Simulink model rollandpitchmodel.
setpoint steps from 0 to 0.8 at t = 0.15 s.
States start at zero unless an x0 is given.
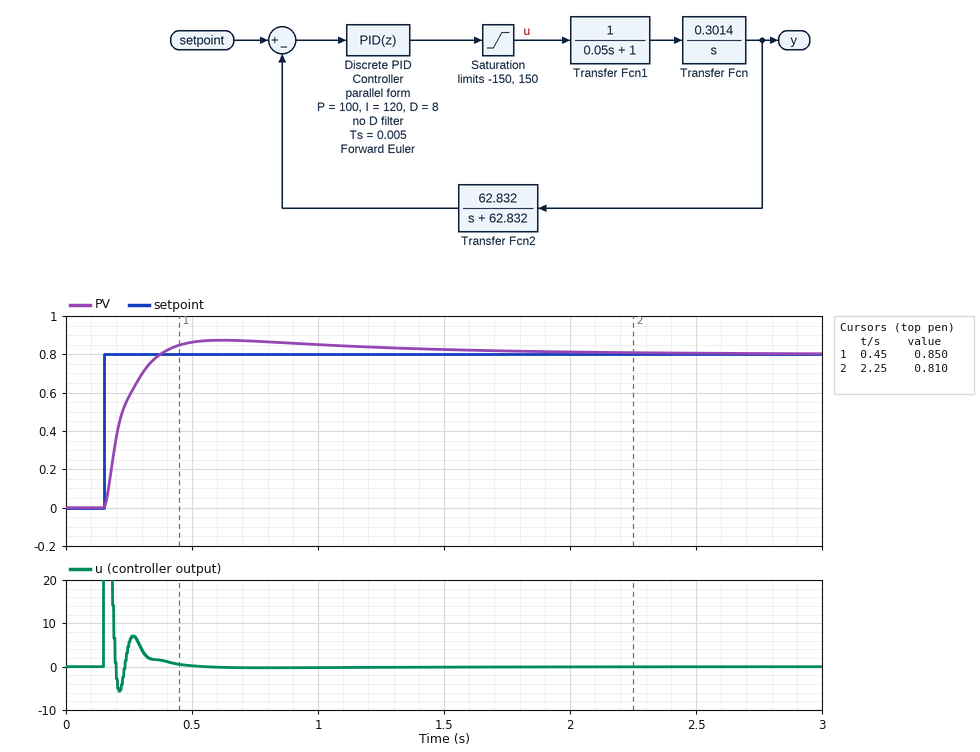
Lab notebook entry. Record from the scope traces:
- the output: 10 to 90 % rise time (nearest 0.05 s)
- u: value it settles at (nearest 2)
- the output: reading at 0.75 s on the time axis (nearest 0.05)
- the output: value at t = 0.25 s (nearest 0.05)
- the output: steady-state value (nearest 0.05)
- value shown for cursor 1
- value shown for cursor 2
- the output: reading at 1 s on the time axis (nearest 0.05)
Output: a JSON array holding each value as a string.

["0.15 s", "0", "0.85", "0.60", "0.80", "0.850", "0.810", "0.85"]
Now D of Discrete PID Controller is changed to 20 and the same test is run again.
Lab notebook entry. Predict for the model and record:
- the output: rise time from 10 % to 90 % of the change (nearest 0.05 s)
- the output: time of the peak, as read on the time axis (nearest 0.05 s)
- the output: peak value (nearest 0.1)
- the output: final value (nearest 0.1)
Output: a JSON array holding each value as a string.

["0.30 s", "1.00 s", "0.9", "0.8"]
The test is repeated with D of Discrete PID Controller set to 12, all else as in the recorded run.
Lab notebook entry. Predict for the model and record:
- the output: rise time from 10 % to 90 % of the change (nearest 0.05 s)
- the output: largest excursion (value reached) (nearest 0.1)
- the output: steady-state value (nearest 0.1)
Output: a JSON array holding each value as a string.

["0.20 s", "0.9", "0.8"]
